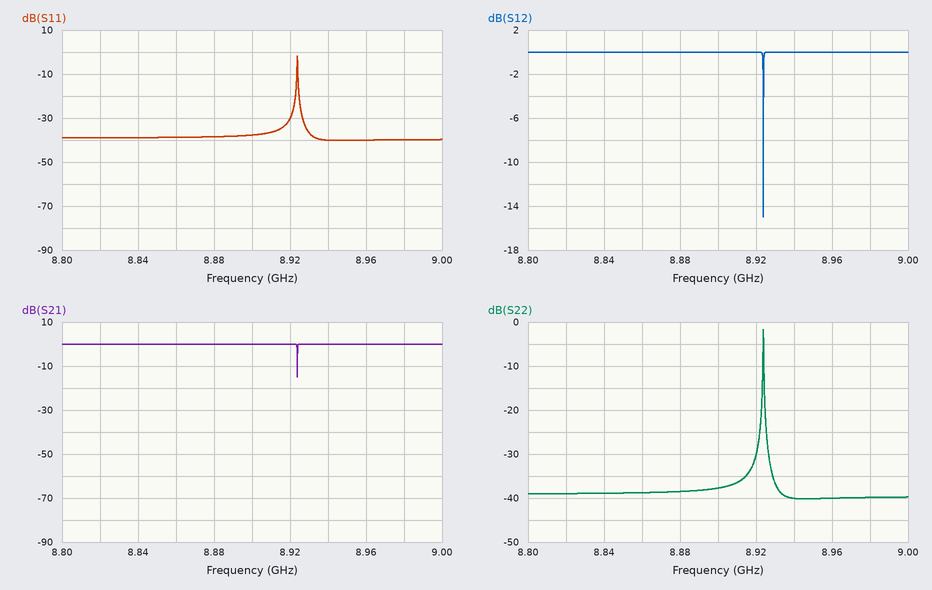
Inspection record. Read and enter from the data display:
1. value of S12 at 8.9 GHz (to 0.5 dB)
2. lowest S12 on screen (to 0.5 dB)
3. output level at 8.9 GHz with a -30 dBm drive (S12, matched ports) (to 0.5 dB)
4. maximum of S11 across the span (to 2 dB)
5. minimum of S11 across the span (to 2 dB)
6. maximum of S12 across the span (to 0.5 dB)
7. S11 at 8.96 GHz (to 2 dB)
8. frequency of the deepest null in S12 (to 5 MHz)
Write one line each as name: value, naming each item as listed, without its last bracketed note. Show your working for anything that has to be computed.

value of S12 at 8.9 GHz: 0.0 dB
lowest S12 on screen: -15.0 dB
output level at 8.9 GHz with a -30 dBm drive (S12, matched ports): -30 dBm + (0.0 dB) = -30.0 dBm
maximum of S11 across the span: -2 dB
minimum of S11 across the span: -40 dB
maximum of S12 across the span: 0.0 dB
S11 at 8.96 GHz: -40 dB
frequency of the deepest null in S12: 8.925 GHz
